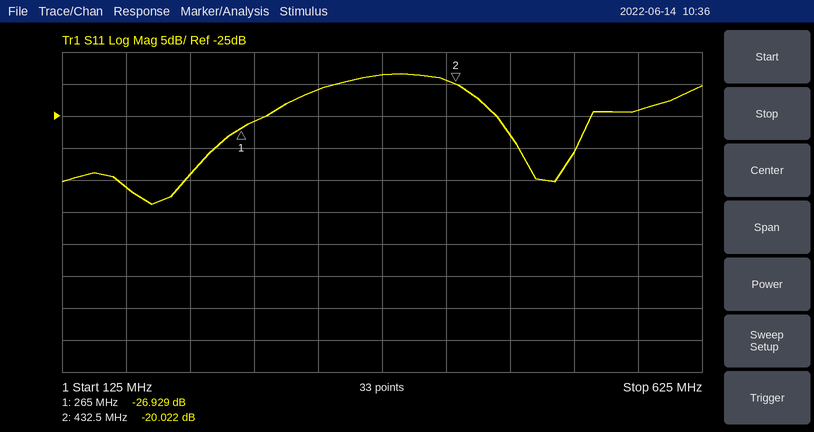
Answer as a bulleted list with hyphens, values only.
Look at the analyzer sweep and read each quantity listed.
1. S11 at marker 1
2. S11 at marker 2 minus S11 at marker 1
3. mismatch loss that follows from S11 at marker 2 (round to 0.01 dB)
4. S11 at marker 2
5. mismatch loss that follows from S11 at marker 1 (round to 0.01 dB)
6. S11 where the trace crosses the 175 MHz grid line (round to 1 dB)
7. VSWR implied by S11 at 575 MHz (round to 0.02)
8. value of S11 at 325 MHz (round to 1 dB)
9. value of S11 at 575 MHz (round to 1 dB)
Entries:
- -26.929 dB
- 6.907 dB
- 0.04 dB
- -20.022 dB
- 0.01 dB
- -36 dB
- 1.14
- -21 dB
- -24 dB
